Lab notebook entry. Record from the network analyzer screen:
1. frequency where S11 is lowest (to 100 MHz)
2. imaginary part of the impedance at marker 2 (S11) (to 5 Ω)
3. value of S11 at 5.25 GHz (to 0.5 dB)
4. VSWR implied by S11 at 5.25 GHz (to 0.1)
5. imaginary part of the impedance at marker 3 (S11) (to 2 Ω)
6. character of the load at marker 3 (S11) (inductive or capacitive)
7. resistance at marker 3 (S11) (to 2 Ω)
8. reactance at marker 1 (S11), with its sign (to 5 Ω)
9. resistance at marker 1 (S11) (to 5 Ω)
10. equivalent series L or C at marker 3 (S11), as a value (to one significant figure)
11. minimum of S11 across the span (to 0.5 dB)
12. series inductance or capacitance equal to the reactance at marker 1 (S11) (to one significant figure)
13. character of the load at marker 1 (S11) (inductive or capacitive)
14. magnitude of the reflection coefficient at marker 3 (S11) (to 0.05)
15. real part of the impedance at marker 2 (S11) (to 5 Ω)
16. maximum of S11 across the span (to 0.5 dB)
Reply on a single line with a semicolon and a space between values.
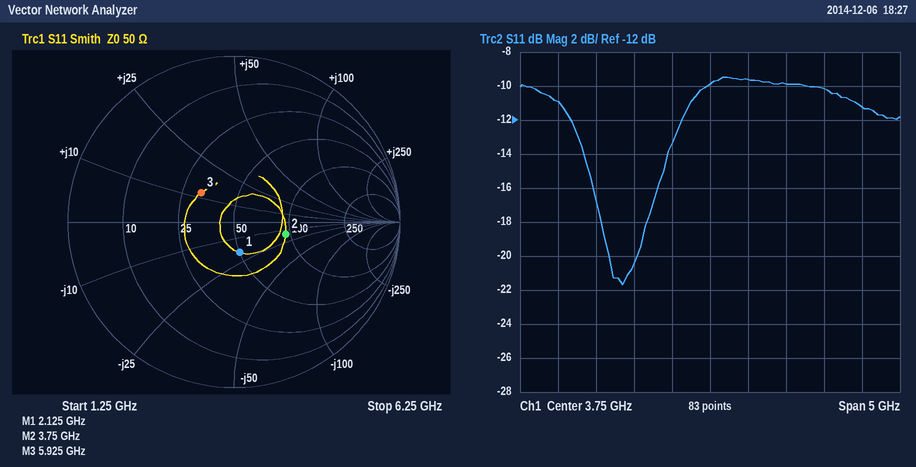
2.6 GHz; -15 Ω; -10.0 dB; 1.9; +12 Ω; inductive; 32 Ω; -20 Ω; 50 Ω; 300 pH; -21.5 dB; 4 pF; capacitive; 0.25; 95 Ω; -9.5 dB
